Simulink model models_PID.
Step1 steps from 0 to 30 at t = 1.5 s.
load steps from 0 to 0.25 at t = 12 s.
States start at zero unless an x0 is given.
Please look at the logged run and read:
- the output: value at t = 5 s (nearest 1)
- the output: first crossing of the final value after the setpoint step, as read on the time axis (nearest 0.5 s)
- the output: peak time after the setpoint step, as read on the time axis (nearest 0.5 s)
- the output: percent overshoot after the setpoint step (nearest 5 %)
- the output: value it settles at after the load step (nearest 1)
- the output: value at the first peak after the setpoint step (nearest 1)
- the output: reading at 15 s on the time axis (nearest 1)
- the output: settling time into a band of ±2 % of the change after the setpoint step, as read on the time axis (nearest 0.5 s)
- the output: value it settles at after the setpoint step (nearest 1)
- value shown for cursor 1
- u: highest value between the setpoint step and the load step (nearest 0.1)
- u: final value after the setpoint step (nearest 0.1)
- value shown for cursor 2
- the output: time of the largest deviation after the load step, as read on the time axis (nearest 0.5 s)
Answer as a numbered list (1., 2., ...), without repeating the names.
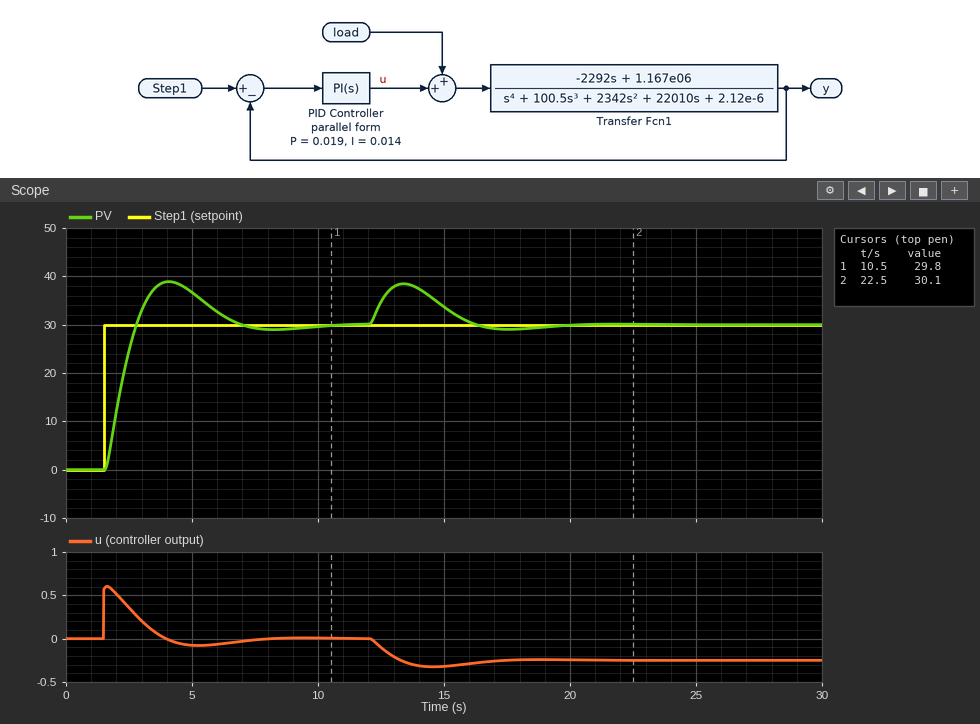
1. 37
2. 3.0 s
3. 4.0 s
4. 30 %
5. 30
6. 39
7. 34
8. 9.5 s
9. 30
10. 29.8
11. 0.6
12. 0.0
13. 30.1
14. 13.5 s
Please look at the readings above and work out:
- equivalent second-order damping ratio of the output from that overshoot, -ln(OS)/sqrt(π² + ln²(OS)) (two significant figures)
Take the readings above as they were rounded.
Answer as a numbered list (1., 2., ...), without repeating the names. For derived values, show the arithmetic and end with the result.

1. ln(0.3) = -1.204; 1.204 / sqrt(9.870 + 1.450) = 0.36
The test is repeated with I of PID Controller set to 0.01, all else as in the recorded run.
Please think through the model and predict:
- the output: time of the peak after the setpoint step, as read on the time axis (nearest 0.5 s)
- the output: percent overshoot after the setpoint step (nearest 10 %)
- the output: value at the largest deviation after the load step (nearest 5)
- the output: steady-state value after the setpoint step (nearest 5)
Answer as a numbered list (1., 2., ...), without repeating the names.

1. 4.5 s
2. 20 %
3. 40
4. 30
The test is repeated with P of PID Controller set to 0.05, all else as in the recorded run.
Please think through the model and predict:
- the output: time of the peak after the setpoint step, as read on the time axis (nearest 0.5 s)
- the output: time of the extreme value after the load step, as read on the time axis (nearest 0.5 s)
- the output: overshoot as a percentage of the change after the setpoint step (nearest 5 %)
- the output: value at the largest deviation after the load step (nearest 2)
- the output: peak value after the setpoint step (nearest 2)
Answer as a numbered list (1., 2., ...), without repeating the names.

1. 3.0 s
2. 13.0 s
3. 10 %
4. 34
5. 32
